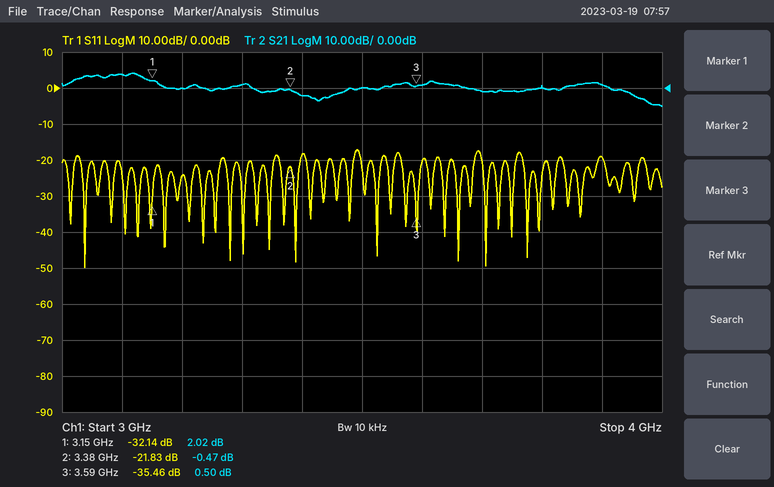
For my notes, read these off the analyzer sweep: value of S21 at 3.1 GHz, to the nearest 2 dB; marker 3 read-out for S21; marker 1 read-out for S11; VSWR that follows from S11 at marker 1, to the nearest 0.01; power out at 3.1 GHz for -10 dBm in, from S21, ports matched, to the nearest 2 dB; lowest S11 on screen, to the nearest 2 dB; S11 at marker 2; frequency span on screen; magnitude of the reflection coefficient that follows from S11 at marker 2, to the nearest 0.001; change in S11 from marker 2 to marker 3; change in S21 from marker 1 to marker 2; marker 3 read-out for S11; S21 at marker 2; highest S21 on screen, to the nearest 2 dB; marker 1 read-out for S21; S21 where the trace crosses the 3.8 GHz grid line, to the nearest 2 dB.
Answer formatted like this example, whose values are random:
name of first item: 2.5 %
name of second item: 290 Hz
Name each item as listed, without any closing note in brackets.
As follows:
value of S21 at 3.1 GHz, to the nearest 2 dB: 4 dB
marker 3 read-out for S21: 0.50 dB
marker 1 read-out for S11: -32.14 dB
VSWR that follows from S11 at marker 1, to the nearest 0.01: 1.05
power out at 3.1 GHz for -10 dBm in, from S21, ports matched, to the nearest 2 dB: -6 dBm
lowest S11 on screen, to the nearest 2 dB: -50 dB
S11 at marker 2: -21.83 dB
frequency span on screen: 1 GHz
magnitude of the reflection coefficient that follows from S11 at marker 2, to the nearest 0.001: 0.081
change in S11 from marker 2 to marker 3: -13.63 dB
change in S21 from marker 1 to marker 2: -2.49 dB
marker 3 read-out for S11: -35.46 dB
S21 at marker 2: -0.47 dB
highest S21 on screen, to the nearest 2 dB: 4 dB
marker 1 read-out for S21: 2.02 dB
S21 where the trace crosses the 3.8 GHz grid line, to the nearest 2 dB: 0 dB
